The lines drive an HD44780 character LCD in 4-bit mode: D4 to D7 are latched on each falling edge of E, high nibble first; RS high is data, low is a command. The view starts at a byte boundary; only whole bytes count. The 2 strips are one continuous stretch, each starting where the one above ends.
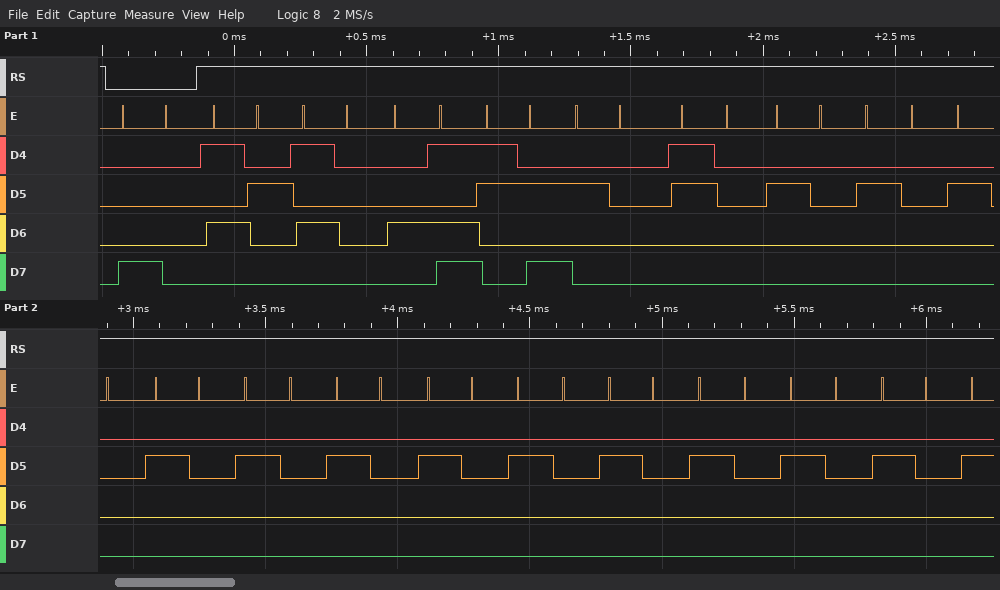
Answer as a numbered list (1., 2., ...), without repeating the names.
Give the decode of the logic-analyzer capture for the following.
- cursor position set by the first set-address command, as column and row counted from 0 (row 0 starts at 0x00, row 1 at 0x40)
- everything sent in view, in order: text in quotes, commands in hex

1. column 0, row 0
2. 0x80 "RPM: 0            "
